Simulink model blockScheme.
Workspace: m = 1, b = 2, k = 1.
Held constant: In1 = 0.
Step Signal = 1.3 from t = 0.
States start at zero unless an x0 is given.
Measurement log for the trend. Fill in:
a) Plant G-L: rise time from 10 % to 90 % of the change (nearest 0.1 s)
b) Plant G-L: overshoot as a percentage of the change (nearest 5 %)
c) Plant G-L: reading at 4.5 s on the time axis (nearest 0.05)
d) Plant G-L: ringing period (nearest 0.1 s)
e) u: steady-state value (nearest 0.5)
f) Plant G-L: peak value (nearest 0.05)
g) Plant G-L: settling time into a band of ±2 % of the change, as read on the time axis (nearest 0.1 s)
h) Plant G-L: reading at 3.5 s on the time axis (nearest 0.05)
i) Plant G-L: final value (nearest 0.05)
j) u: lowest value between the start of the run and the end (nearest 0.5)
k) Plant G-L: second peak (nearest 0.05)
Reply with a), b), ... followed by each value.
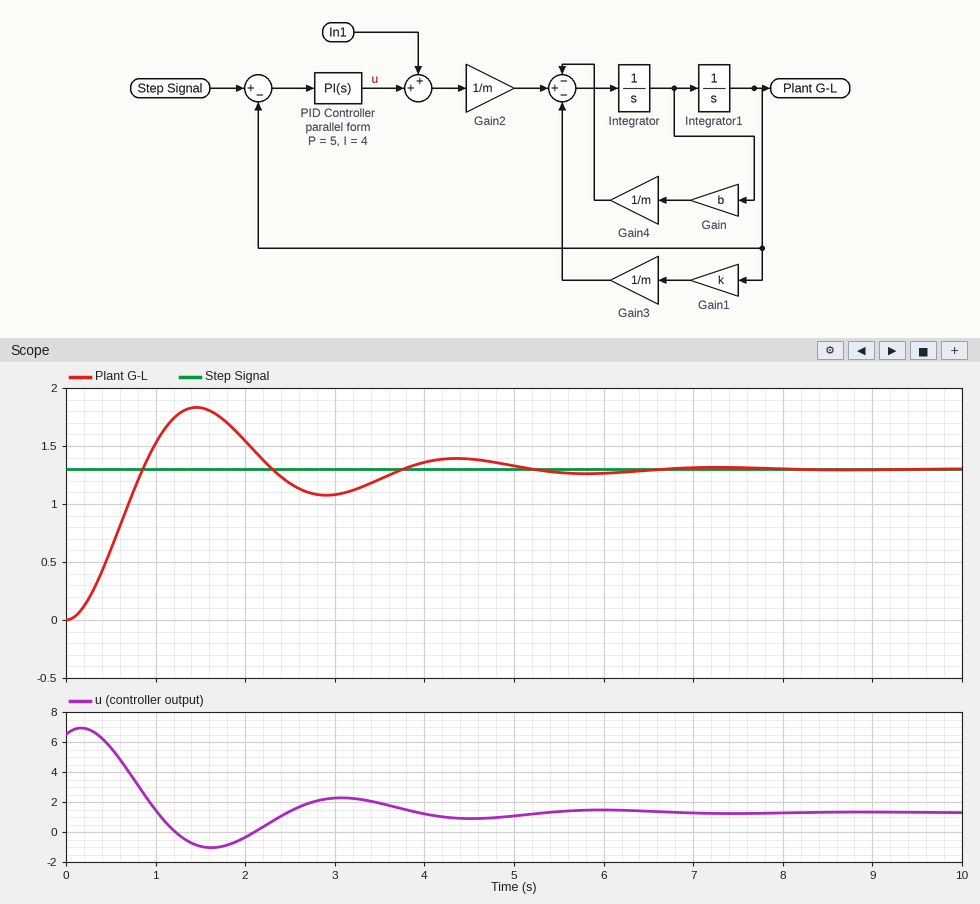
a) 0.6 s
b) 40 %
c) 1.40
d) 2.9 s
e) 1.5
f) 1.85
g) 6.2 s
h) 1.20
i) 1.30
j) -1.0
k) 1.40
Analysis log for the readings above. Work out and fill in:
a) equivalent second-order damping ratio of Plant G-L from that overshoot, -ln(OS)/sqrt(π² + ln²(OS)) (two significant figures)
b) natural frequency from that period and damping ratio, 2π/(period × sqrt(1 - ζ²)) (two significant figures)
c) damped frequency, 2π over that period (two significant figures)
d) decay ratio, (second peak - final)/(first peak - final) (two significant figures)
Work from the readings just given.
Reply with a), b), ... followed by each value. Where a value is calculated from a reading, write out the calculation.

a) ln(0.4) = -0.916; 0.916 / sqrt(9.870 + 0.840) = 0.28
b) 2π / (2.9 × sqrt(1 - 0.28²)) = 2.3 rad/s
c) 2π / 2.9 = 2.2 rad/s
d) (1.4 - 1.3) / (1.85 - 1.3) = 0.18
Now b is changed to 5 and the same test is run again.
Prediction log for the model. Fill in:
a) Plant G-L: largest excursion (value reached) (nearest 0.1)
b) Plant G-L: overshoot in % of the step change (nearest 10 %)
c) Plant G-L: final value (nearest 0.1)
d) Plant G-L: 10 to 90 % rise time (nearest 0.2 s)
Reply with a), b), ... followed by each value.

a) 1.6
b) 20 %
c) 1.3
d) 1.0 s
